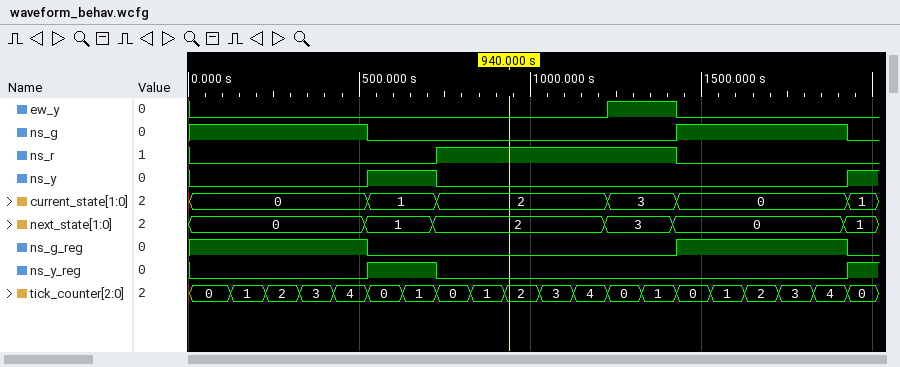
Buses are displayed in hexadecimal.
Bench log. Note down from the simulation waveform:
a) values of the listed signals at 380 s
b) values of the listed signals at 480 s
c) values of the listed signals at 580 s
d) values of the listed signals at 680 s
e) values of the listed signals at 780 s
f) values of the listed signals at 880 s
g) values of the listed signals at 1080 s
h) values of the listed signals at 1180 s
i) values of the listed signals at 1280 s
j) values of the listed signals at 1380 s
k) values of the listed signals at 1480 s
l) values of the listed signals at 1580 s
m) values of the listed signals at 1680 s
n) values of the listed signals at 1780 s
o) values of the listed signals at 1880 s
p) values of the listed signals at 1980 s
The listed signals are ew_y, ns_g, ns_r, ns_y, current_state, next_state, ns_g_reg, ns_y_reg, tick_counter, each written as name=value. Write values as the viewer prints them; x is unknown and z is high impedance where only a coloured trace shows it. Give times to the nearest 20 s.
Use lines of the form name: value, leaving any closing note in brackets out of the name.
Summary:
values of the listed signals at 380 s: ew_y=0, ns_g=1, ns_r=0, ns_y=0, current_state=0, next_state=0, ns_g_reg=1, ns_y_reg=0, tick_counter=3
values of the listed signals at 480 s: ew_y=0, ns_g=1, ns_r=0, ns_y=0, current_state=0, next_state=0, ns_g_reg=1, ns_y_reg=0, tick_counter=4
values of the listed signals at 580 s: ew_y=0, ns_g=0, ns_r=0, ns_y=1, current_state=1, next_state=1, ns_g_reg=0, ns_y_reg=1, tick_counter=0
values of the listed signals at 680 s: ew_y=0, ns_g=0, ns_r=0, ns_y=1, current_state=1, next_state=1, ns_g_reg=0, ns_y_reg=1, tick_counter=1
values of the listed signals at 780 s: ew_y=0, ns_g=0, ns_r=1, ns_y=0, current_state=2, next_state=2, ns_g_reg=0, ns_y_reg=0, tick_counter=0
values of the listed signals at 880 s: ew_y=0, ns_g=0, ns_r=1, ns_y=0, current_state=2, next_state=2, ns_g_reg=0, ns_y_reg=0, tick_counter=1
values of the listed signals at 1080 s: ew_y=0, ns_g=0, ns_r=1, ns_y=0, current_state=2, next_state=2, ns_g_reg=0, ns_y_reg=0, tick_counter=3
values of the listed signals at 1180 s: ew_y=0, ns_g=0, ns_r=1, ns_y=0, current_state=2, next_state=2, ns_g_reg=0, ns_y_reg=0, tick_counter=4
values of the listed signals at 1280 s: ew_y=1, ns_g=0, ns_r=1, ns_y=0, current_state=3, next_state=3, ns_g_reg=0, ns_y_reg=0, tick_counter=0
values of the listed signals at 1380 s: ew_y=1, ns_g=0, ns_r=1, ns_y=0, current_state=3, next_state=3, ns_g_reg=0, ns_y_reg=0, tick_counter=1
values of the listed signals at 1480 s: ew_y=0, ns_g=1, ns_r=0, ns_y=0, current_state=0, next_state=0, ns_g_reg=1, ns_y_reg=0, tick_counter=0
values of the listed signals at 1580 s: ew_y=0, ns_g=1, ns_r=0, ns_y=0, current_state=0, next_state=0, ns_g_reg=1, ns_y_reg=0, tick_counter=1
values of the listed signals at 1680 s: ew_y=0, ns_g=1, ns_r=0, ns_y=0, current_state=0, next_state=0, ns_g_reg=1, ns_y_reg=0, tick_counter=2
values of the listed signals at 1780 s: ew_y=0, ns_g=1, ns_r=0, ns_y=0, current_state=0, next_state=0, ns_g_reg=1, ns_y_reg=0, tick_counter=3
values of the listed signals at 1880 s: ew_y=0, ns_g=1, ns_r=0, ns_y=0, current_state=0, next_state=0, ns_g_reg=1, ns_y_reg=0, tick_counter=4
values of the listed signals at 1980 s: ew_y=0, ns_g=0, ns_r=0, ns_y=1, current_state=1, next_state=1, ns_g_reg=0, ns_y_reg=1, tick_counter=0
